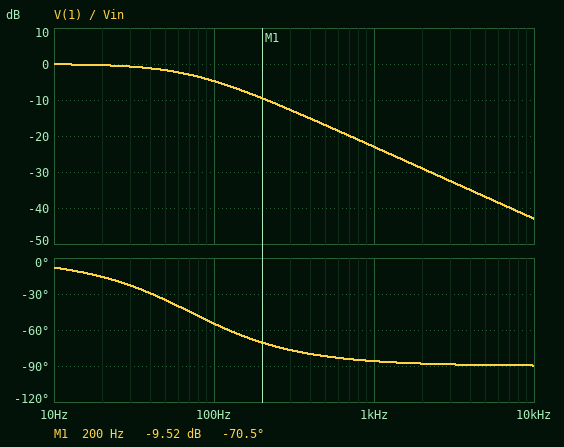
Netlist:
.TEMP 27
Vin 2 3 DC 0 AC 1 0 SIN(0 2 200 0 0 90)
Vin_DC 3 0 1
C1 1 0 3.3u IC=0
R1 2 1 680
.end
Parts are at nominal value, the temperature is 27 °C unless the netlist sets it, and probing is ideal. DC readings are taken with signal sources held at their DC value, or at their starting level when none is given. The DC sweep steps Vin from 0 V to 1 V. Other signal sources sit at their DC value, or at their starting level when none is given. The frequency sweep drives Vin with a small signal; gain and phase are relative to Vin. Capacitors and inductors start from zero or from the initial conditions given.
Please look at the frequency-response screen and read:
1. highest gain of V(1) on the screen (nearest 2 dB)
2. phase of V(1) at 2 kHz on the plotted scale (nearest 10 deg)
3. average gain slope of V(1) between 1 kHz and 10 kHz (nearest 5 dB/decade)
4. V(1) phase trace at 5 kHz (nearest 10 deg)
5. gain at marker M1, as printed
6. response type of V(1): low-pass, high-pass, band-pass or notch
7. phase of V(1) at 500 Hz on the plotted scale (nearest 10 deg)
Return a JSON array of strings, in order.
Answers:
["0 dB", "-90 deg", "-20 dB/decade", "-90 deg", "-9.52 dB", "low-pass", "-80 deg"]
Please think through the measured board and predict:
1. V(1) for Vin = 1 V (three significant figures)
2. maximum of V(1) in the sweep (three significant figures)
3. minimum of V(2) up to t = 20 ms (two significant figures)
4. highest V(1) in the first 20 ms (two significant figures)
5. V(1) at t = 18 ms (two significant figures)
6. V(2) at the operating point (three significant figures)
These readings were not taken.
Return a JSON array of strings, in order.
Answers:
["2.00 V", "2.00 V", "-1.0 V", "1.7 V", "450 mV", "1.00 V"]
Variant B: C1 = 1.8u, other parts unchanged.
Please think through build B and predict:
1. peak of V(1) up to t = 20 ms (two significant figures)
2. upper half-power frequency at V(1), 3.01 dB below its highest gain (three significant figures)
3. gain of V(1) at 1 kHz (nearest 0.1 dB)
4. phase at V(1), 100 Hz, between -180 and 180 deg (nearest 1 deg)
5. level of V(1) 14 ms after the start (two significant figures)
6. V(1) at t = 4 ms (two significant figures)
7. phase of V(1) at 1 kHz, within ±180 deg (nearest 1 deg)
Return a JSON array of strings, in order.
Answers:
["2.1 V", "130 Hz", "-17.8 dB", "-38 deg", "310 mV", "250 mV", "-83 deg"]
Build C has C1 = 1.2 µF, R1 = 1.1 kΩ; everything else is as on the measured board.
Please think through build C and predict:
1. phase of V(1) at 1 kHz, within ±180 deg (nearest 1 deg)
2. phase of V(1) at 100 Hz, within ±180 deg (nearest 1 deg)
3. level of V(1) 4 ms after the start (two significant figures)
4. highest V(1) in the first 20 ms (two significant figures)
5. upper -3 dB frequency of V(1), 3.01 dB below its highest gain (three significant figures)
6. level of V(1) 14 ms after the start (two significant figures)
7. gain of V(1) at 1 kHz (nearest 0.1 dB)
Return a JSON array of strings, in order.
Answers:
["-83 deg", "-40 deg", "250 mV", "2.0 V", "121 Hz", "320 mV", "-18.4 dB"]
